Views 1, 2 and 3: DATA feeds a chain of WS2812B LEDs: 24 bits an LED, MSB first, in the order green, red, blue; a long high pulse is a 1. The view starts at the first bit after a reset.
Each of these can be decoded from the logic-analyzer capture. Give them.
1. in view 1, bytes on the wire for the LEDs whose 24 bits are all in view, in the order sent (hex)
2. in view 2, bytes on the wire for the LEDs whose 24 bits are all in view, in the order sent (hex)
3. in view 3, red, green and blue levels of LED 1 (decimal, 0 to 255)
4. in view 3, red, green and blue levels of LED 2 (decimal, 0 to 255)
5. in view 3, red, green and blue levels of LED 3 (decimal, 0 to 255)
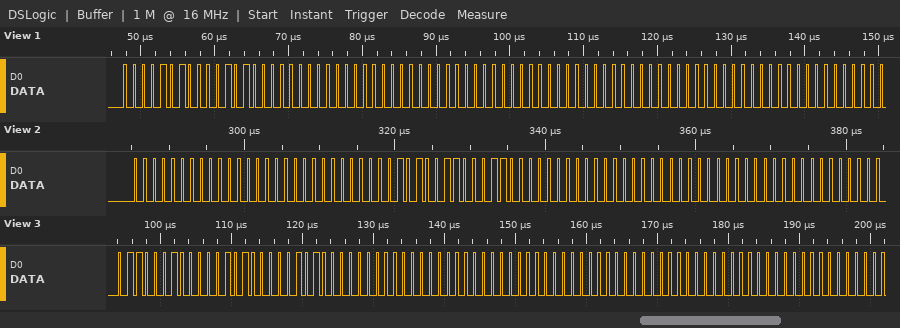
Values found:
0A 14 00 00 00 00 00 00 00
00 00 00 0A 63 00 00 00 00
10, 98, 10
0, 0, 0
0, 0, 0
